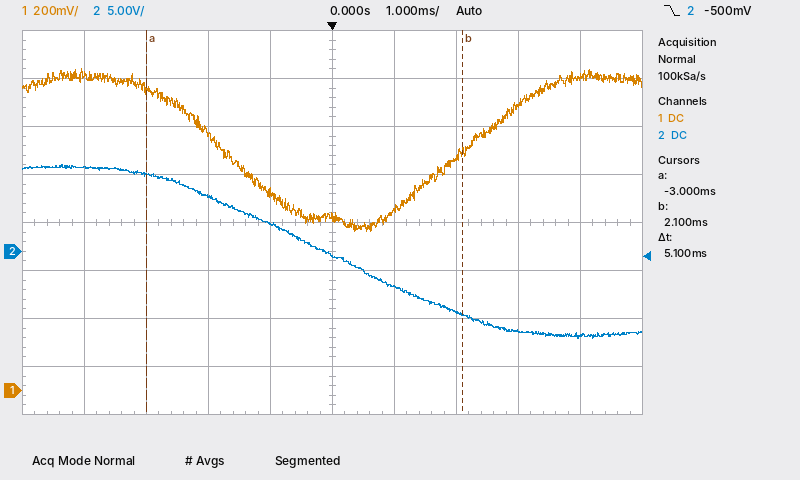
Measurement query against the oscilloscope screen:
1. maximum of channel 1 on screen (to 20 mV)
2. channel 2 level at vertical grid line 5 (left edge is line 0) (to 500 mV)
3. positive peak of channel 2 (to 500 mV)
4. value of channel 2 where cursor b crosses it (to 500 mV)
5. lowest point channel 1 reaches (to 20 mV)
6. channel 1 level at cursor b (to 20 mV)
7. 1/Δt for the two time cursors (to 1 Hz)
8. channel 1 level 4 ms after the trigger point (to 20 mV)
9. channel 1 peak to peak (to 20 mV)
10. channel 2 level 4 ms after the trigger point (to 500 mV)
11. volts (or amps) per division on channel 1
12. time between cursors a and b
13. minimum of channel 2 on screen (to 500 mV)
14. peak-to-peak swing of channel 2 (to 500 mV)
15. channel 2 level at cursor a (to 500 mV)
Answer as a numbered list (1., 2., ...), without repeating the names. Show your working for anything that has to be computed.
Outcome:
1. 1.34 V
2. -500 mV
3. 9.0 V
4. -6.5 V
5. 660 mV
6. 1.00 V
7. 1 / 5.1 ms ≈ 196 Hz
8. 1.30 V
9. 1.34 V − (660 mV) = 680 mV
10. -9.0 V
11. 200 mV
12. 5.1 ms
13. -9.0 V
14. 9.0 V − (-9.0 V) = 18.0 V
15. 8.0 V
